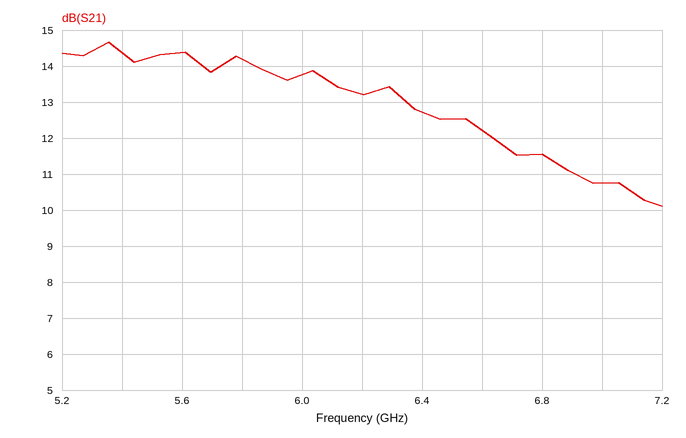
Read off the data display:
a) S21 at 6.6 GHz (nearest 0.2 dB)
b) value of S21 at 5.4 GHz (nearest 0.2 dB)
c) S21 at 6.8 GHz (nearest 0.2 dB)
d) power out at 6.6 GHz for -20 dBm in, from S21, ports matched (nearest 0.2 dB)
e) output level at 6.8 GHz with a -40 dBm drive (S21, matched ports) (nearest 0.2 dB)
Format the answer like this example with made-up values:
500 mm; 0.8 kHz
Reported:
12.2 dB; 14.4 dB; 11.6 dB; -7.8 dBm; -28.4 dBm
